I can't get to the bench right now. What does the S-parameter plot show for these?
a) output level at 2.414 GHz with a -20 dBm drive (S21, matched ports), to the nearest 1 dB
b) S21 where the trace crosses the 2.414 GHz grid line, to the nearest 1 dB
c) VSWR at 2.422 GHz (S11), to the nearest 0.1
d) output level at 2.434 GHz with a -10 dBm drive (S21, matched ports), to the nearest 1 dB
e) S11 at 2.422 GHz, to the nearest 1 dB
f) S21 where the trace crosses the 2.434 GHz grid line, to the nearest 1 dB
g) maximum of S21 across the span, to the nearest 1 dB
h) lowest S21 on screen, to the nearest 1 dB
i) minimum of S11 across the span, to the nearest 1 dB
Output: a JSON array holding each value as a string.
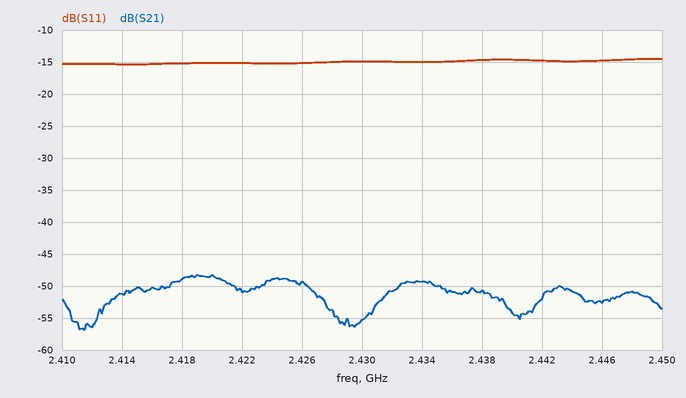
["-71 dBm", "-51 dB", "1.4", "-59 dBm", "-15 dB", "-49 dB", "-48 dB", "-57 dB", "-15 dB"]
